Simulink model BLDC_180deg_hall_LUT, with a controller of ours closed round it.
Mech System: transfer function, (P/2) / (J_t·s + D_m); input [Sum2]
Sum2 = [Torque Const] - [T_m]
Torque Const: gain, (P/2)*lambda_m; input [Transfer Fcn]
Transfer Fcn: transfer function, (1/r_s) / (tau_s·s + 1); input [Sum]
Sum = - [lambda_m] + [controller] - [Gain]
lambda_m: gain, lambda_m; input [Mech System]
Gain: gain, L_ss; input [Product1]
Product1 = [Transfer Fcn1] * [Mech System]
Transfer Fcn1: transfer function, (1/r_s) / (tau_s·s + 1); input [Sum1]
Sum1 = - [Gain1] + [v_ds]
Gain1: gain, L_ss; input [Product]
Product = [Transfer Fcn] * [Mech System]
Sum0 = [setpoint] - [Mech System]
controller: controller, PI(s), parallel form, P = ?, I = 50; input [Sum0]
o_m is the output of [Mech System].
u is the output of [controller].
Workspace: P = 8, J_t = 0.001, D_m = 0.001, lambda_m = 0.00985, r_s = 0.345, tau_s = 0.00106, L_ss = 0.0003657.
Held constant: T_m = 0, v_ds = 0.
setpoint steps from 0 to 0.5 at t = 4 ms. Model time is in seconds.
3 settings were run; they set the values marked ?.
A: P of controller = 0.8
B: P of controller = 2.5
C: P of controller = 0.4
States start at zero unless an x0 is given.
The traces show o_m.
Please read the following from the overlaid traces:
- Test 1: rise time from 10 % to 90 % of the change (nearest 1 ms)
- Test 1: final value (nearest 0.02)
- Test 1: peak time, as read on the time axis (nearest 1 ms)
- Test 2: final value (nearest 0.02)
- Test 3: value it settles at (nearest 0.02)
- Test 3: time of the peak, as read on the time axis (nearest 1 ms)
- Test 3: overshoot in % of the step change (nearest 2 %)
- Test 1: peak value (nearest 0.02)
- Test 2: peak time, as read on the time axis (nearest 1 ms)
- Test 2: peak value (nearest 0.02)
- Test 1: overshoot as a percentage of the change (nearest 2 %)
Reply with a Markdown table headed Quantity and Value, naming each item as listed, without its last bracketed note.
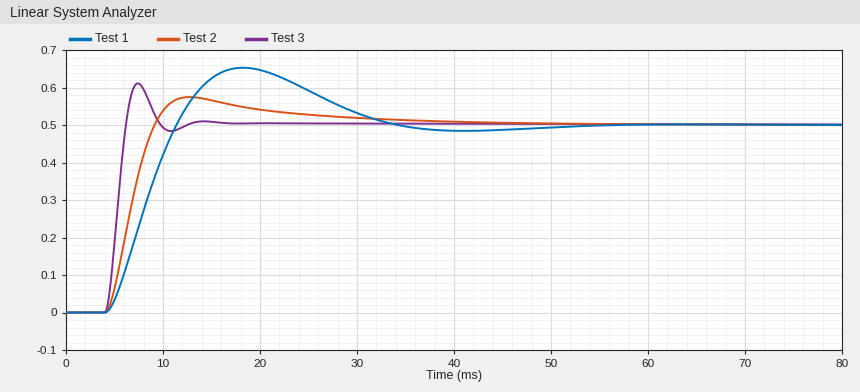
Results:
| Quantity | Value |
|---|---|
| Test 1: rise time from 10 % to 90 % of the change | 5 ms |
| Test 1: final value | 0.50 |
| Test 1: peak time, as read on the time axis | 18 ms |
| Test 2: final value | 0.50 |
| Test 3: value it settles at | 0.50 |
| Test 3: time of the peak, as read on the time axis | 7 ms |
| Test 3: overshoot in % of the step change | 22 % |
| Test 1: peak value | 0.66 |
| Test 2: peak time, as read on the time axis | 13 ms |
| Test 2: peak value | 0.58 |
| Test 1: overshoot as a percentage of the change | 30 % |
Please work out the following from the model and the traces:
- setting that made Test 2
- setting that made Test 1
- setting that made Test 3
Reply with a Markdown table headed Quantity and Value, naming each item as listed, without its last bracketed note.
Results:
| Quantity | Value |
|---|---|
| setting that made Test 2 | A |
| setting that made Test 1 | C |
| setting that made Test 3 | B |
